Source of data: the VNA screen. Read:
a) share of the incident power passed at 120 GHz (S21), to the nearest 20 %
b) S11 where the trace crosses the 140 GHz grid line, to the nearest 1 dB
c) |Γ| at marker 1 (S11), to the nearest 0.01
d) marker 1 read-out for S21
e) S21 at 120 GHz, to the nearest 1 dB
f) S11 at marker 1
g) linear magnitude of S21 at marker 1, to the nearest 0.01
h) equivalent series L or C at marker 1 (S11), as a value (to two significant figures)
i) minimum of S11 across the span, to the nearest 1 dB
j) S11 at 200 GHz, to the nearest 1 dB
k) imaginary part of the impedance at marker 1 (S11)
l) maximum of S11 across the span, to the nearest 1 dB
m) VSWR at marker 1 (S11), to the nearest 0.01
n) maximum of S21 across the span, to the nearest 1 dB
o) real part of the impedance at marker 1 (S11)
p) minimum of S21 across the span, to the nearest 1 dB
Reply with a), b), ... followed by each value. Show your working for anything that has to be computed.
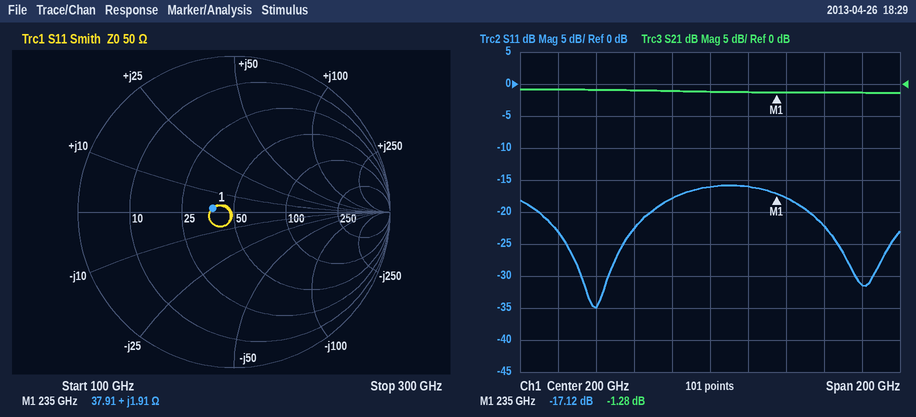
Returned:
a) 10^(-1/10) ≈ 79.4 %, so 80 % to the nearest 20 %
b) -35 dB
c) 0.14
d) -1.28 dB
e) -1 dB
f) -17.12 dB
g) 10^(-1.28/20) ≈ 0.86
h) L = 1.91 Ω/(2π × 235 GHz) ≈ 1.3 pH
i) -35 dB
j) -16 dB
k) +1.91 Ω
l) -16 dB
m) (1 + 0.1393)/(1 − 0.1393) ≈ 1.32
n) -1 dB
o) 37.91 Ω
p) -1 dB
